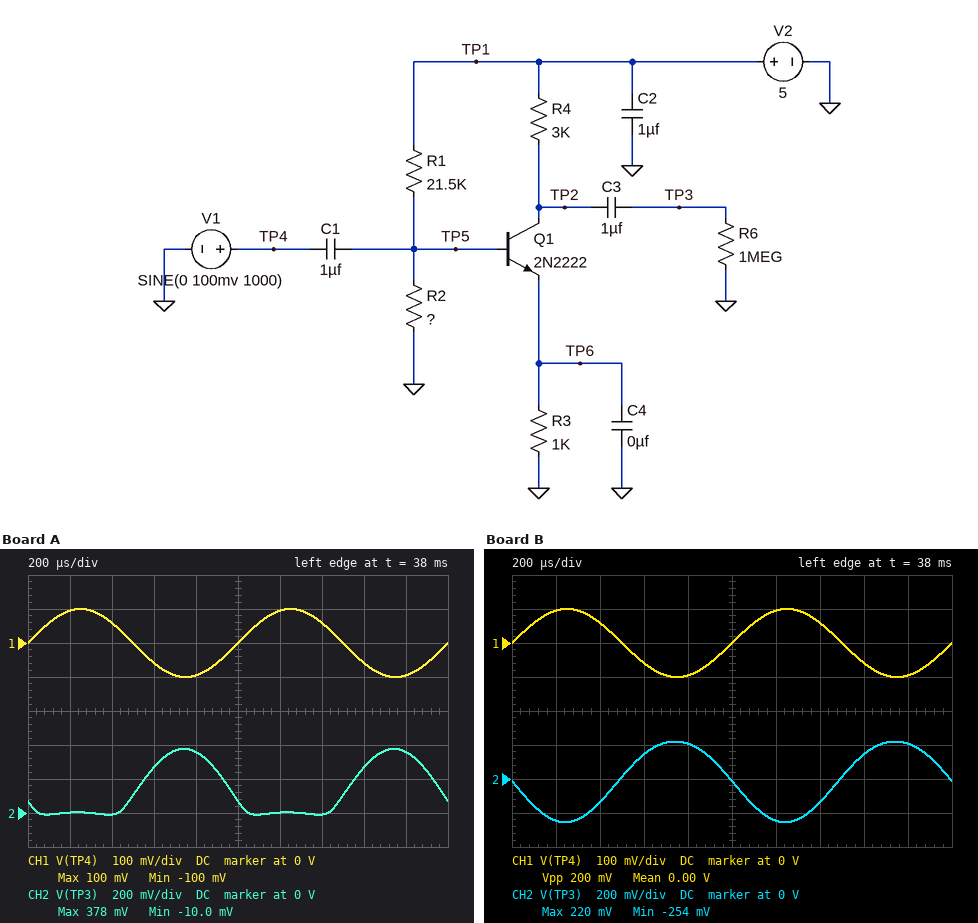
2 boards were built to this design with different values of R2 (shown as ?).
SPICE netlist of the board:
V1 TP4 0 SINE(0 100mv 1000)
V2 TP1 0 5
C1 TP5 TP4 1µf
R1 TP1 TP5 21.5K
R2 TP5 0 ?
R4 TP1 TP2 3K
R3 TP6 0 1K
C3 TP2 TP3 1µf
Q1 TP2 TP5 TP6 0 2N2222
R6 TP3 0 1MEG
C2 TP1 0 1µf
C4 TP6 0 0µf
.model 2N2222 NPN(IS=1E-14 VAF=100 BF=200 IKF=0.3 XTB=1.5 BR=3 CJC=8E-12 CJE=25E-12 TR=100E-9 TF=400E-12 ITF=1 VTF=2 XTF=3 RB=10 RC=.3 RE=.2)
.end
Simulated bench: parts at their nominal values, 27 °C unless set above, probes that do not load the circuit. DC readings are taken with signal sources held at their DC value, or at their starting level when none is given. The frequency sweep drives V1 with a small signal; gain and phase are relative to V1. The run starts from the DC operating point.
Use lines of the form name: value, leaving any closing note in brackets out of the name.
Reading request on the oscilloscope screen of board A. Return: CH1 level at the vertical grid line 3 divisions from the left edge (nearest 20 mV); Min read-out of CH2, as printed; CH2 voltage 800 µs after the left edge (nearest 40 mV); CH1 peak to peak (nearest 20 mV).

CH1 level at the vertical grid line 3 divisions from the left edge: -60 mV
Min read-out of CH2, as printed: -10.0 mV
CH2 voltage 800 µs after the left edge: 360 mV
CH1 peak to peak: 200 mV
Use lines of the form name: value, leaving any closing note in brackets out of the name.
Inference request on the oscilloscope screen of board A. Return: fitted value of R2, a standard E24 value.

fitted value of R2, a standard E24 value: 15 kΩ
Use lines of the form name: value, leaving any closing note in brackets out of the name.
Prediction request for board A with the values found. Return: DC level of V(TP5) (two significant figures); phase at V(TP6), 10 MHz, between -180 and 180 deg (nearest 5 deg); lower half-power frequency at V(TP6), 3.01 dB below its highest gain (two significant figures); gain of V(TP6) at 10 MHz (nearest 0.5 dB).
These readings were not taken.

DC level of V(TP5): 1.9 V
phase at V(TP6), 10 MHz, between -180 and 180 deg: 0 deg
lower half-power frequency at V(TP6), 3.01 dB below its highest gain: 150 Hz
gain of V(TP6) at 10 MHz: -0.5 dB
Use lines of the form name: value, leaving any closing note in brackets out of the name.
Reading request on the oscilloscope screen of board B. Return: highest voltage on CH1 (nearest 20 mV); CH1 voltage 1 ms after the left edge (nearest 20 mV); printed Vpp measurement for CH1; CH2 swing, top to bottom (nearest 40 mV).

highest voltage on CH1: 100 mV
CH1 voltage 1 ms after the left edge: 0 V
printed Vpp measurement for CH1: 200 mV
CH2 swing, top to bottom: 480 mV
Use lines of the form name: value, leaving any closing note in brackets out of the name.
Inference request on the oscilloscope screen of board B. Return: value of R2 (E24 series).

value of R2: 3.6 kΩ
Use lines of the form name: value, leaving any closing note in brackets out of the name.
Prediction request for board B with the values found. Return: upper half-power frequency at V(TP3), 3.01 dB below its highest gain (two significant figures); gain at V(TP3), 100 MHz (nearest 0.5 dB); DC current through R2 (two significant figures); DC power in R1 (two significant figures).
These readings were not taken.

upper half-power frequency at V(TP3), 3.01 dB below its highest gain: 17 MHz
gain at V(TP3), 100 MHz: 0.5 dB
DC current through R2: 200 µA
DC power in R1: 850 µW
